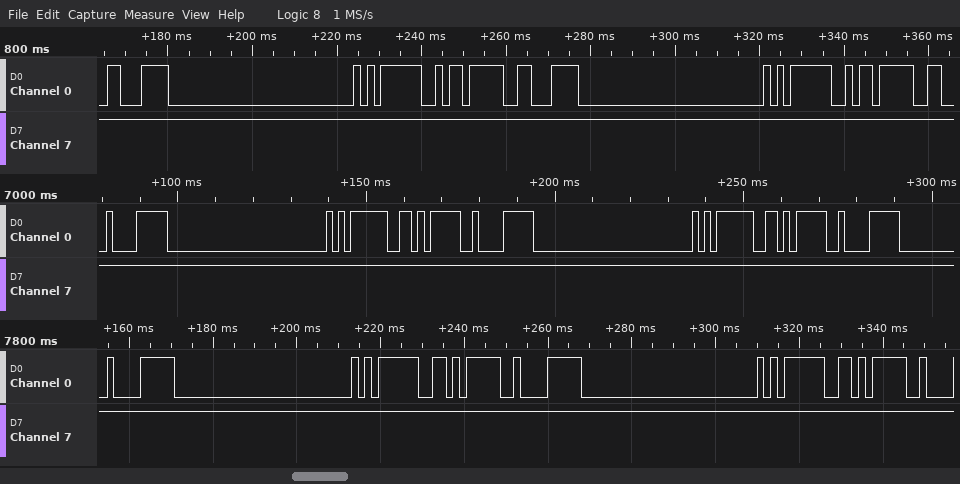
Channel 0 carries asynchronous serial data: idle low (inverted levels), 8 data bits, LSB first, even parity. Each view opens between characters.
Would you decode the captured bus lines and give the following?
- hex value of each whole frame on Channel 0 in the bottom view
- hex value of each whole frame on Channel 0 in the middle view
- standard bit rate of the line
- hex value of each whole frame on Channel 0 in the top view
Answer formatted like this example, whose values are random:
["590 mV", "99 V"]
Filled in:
["0F, 05, 0A, 0F, 05, 0A", "0F, 05, 0A, 0F, 05, 0A, 0F", "600 baud", "0E, 05, 09, 0E, 05, 09"]
